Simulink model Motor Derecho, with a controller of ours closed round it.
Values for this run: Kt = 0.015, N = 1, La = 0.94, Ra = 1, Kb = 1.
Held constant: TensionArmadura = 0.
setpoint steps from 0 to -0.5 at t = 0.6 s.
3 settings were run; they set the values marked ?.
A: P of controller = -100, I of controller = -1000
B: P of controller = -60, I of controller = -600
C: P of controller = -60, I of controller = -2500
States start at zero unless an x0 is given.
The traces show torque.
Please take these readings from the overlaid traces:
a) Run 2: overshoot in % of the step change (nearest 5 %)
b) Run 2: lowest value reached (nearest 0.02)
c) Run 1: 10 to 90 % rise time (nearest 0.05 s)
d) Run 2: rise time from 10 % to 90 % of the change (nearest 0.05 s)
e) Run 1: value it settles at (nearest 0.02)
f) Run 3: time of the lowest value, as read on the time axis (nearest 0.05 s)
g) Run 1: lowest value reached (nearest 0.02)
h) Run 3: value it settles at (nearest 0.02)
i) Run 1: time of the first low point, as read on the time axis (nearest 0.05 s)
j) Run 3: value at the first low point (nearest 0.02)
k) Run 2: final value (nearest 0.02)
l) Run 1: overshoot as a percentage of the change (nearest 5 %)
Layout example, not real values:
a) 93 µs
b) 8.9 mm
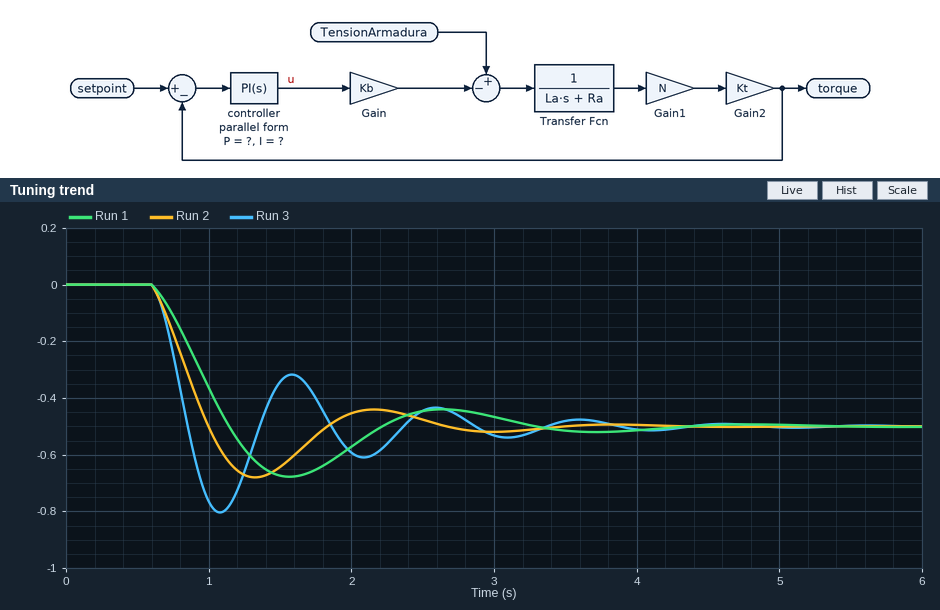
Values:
a) 35 %
b) -0.68
c) 0.40 s
d) 0.30 s
e) -0.50
f) 1.10 s
g) -0.68
h) -0.50
i) 1.55 s
j) -0.80
k) -0.50
l) 35 %
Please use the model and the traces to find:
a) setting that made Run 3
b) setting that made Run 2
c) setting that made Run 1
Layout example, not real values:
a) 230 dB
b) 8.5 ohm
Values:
a) C
b) A
c) B
